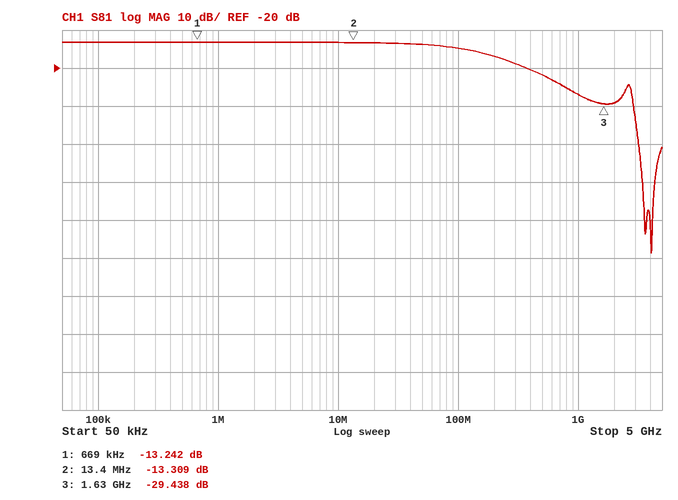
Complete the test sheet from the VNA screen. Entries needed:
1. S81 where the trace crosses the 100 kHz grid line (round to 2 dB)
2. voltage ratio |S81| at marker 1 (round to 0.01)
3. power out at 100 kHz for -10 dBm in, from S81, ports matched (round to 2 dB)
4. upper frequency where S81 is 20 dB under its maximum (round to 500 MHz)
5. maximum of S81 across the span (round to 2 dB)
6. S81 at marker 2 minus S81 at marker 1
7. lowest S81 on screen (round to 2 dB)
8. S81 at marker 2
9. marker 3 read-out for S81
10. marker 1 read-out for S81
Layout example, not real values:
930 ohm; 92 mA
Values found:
-14 dB; 0.22; -24 dBm; 3.0 GHz; -14 dB; -0.067 dB; -68 dB; -13.309 dB; -29.438 dB; -13.242 dB
